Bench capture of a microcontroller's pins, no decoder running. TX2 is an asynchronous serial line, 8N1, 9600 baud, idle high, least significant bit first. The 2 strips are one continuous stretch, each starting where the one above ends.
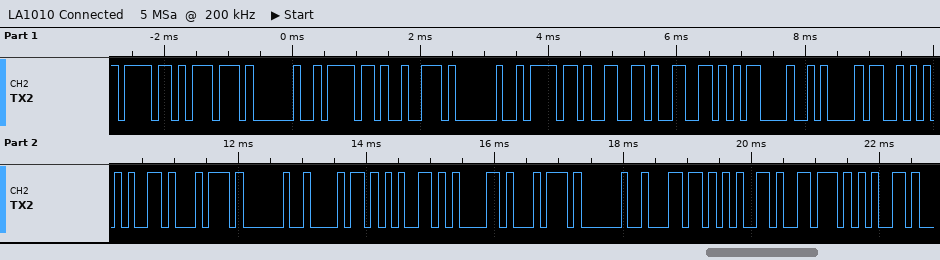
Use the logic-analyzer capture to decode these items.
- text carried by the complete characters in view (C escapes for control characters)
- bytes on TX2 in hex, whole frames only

"ow or off\r\nSet heat leve"
0x6F 0x77 0x20 0x6F 0x72 0x20 0x6F 0x66 0x66 0x0D 0x0A 0x53 0x65 0x74 0x20 0x68 0x65 0x61 0x74 0x20 0x6C 0x65 0x76 0x65
